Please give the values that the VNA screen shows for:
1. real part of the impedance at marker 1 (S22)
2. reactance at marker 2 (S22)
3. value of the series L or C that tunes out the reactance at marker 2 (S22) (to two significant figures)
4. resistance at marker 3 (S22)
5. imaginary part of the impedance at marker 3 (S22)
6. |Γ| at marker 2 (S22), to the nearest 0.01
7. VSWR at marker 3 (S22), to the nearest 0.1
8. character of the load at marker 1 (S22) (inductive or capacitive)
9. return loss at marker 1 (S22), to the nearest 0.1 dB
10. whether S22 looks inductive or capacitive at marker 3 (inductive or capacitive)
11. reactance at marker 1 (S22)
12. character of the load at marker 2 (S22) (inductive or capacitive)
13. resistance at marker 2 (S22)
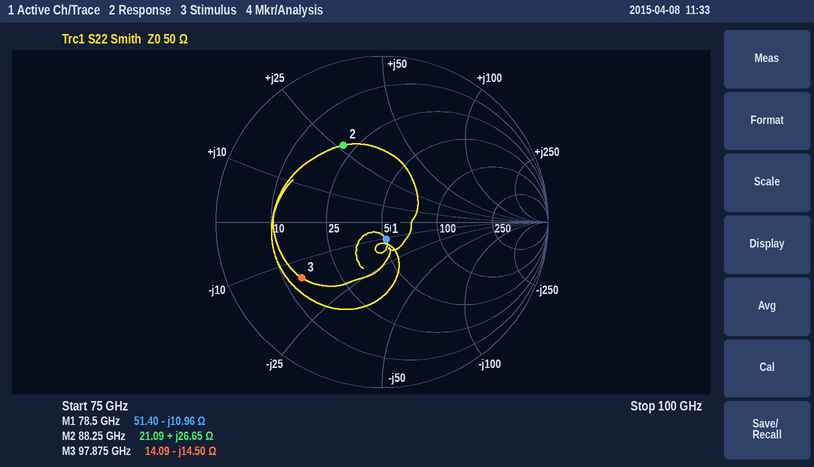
51.40 Ω
+26.65 Ω
68 fF
14.09 Ω
-14.50 Ω
0.52
3.9
capacitive
19.3 dB
capacitive
-10.96 Ω
inductive
21.09 Ω
